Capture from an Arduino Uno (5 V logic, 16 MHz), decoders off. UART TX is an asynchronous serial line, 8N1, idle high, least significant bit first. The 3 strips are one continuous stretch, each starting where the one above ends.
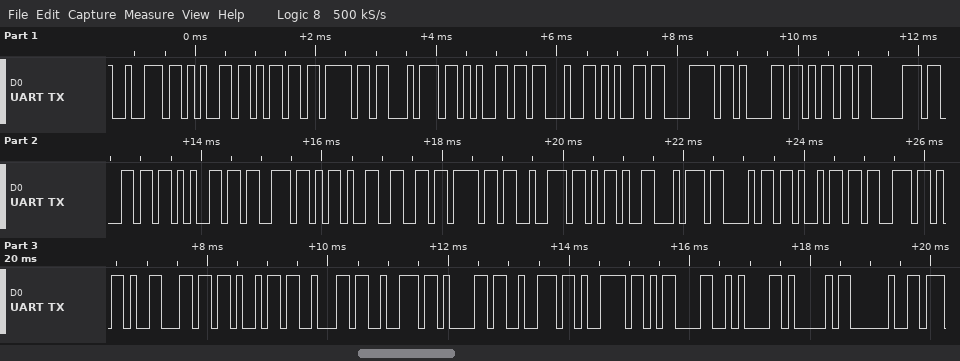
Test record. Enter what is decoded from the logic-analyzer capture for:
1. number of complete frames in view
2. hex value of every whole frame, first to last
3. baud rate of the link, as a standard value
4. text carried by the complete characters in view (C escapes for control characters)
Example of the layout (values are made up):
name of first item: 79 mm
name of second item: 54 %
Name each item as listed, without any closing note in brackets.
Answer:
number of complete frames in view: 36
hex value of every whole frame, first to last: 72 65 6D 6F 74 65 23 65 78 61 6D 70 6C 65 73 2D 66 6F 72 2D 74 68 69 73 2D 6C 69 62 72 61 72 79 0D 0A 41 20
baud rate of the link, as a standard value: 9600 baud
text carried by the complete characters in view: "remote#examples-for-this-library\r\nA "
